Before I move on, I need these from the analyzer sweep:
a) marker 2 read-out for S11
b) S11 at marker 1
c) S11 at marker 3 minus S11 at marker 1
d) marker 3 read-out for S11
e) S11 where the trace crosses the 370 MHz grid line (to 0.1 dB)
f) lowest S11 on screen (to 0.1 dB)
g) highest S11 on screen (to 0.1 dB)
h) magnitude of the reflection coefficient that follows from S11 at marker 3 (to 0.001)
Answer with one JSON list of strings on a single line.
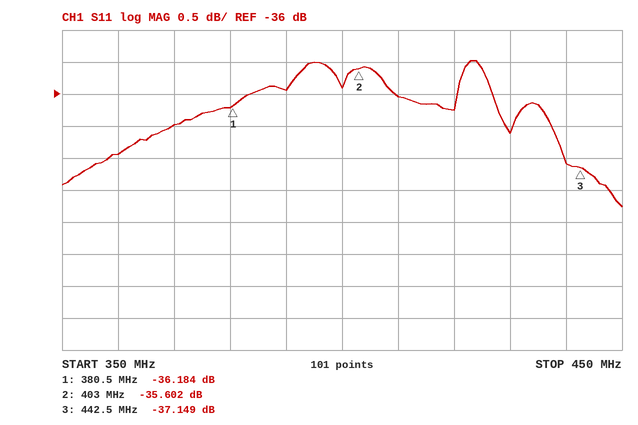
["-35.602 dB", "-36.184 dB", "-0.965 dB", "-37.149 dB", "-36.5 dB", "-37.8 dB", "-35.5 dB", "0.014"]
